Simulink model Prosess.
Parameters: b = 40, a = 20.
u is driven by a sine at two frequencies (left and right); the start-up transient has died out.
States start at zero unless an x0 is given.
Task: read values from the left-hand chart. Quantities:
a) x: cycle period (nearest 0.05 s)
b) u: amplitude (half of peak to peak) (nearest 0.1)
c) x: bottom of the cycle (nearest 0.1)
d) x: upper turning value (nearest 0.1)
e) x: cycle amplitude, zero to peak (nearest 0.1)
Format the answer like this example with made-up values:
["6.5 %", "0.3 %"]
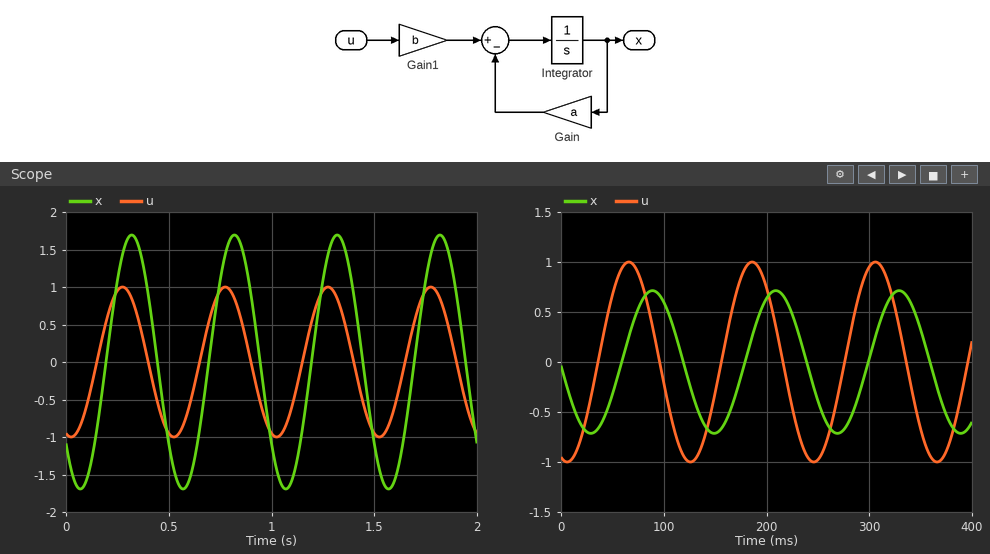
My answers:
["0.50 s", "1.0", "-1.7", "1.7", "1.7"]
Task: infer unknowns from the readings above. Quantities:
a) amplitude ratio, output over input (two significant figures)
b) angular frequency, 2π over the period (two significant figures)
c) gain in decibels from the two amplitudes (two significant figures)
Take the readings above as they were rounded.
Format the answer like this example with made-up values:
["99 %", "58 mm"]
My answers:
["1.7", "13 rad/s", "4.6 dB"]
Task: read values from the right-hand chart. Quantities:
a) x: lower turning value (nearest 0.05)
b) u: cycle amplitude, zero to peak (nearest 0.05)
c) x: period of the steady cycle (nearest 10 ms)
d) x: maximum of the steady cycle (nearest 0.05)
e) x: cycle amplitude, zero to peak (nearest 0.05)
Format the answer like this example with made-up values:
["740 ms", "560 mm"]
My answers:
["-0.70", "1.00", "120 ms", "0.70", "0.70"]
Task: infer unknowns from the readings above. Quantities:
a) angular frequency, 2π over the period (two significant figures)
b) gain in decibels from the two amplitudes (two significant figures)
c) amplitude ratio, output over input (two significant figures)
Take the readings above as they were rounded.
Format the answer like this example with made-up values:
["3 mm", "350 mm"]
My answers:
["0.052 rad/ms", "-3.1 dB", "0.70"]
